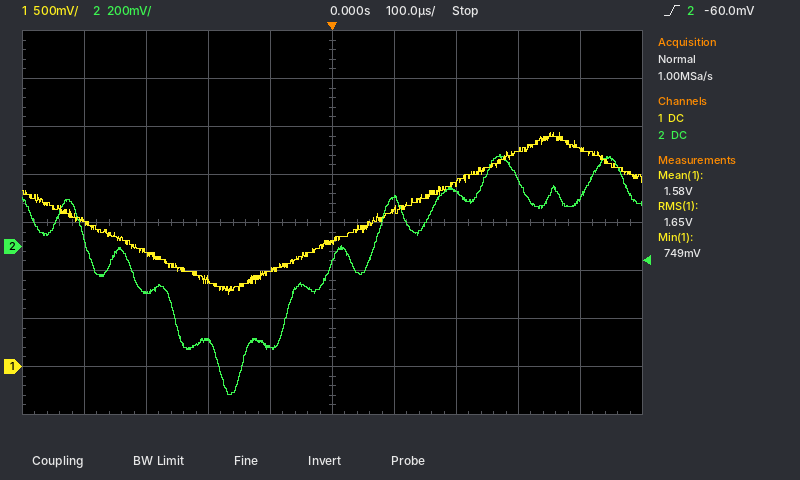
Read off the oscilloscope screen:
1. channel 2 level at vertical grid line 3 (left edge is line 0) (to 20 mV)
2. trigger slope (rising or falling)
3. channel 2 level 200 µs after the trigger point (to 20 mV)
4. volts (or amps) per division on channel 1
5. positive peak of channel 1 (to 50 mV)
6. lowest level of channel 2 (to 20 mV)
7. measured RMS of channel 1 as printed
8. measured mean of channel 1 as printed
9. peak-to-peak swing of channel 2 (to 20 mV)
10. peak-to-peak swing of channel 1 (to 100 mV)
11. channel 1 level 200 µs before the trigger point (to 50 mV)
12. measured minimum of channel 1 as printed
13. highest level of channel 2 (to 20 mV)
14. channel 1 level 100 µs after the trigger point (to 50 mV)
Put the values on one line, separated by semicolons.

-400 mV; rising; 220 mV; 500 mV; 2.45 V; -620 mV; 1.65 V; 1.58 V; 1.00 V; 1.70 V; 900 mV; 749 mV; 380 mV; 1.65 V
